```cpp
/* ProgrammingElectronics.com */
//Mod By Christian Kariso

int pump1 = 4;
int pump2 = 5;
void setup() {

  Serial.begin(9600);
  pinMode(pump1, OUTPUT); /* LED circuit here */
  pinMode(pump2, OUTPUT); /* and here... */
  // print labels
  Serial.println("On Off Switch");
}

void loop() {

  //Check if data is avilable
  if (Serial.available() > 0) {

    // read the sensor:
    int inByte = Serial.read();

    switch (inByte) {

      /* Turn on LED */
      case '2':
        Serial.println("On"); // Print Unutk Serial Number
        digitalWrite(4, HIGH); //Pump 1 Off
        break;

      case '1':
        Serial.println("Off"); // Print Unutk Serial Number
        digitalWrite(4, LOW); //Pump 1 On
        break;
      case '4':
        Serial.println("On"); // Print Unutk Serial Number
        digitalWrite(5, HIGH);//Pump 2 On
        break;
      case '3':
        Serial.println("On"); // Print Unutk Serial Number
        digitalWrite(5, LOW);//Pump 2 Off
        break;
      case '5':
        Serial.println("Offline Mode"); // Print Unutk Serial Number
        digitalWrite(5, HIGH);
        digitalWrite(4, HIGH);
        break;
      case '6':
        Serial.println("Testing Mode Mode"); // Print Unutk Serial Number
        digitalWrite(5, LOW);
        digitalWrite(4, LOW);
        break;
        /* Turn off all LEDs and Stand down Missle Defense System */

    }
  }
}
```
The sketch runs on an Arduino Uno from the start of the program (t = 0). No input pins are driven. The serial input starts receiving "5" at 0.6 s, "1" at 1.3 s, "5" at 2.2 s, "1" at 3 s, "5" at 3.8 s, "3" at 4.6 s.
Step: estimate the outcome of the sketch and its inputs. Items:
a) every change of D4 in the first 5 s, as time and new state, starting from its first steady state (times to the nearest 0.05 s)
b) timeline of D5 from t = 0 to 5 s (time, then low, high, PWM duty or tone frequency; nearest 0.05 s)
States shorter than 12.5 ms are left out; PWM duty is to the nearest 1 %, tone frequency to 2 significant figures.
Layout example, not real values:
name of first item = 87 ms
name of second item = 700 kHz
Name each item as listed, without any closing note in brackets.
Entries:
every change of D4 in the first 5 s, as time and new state, starting from its first steady state = 0 s low; 0.6 s high; 1.3 s low; 2.2 s high; 3 s low; 3.8 s high
timeline of D5 from t = 0 to 5 s = 0 s low; 0.6 s high; 4.6 s low
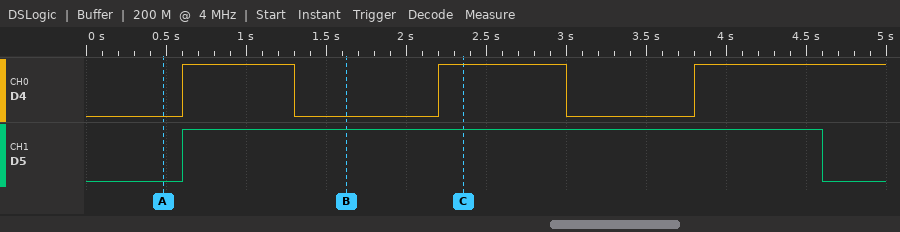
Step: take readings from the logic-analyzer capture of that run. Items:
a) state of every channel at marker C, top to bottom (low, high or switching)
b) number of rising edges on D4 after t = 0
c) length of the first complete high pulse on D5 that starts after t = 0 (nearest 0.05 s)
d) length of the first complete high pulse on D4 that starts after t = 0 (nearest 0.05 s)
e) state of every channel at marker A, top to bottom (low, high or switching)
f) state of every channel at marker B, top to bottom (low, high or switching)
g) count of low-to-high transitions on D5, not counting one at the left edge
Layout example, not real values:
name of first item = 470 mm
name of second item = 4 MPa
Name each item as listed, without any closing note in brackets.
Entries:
state of every channel at marker C, top to bottom = D4 high, D5 high
number of rising edges on D4 after t = 0 = 3
length of the first complete high pulse on D5 that starts after t = 0 = 4.00 s
length of the first complete high pulse on D4 that starts after t = 0 = 0.70 s
state of every channel at marker A, top to bottom = D4 low, D5 low
state of every channel at marker B, top to bottom = D4 low, D5 high
count of low-to-high transitions on D5, not counting one at the left edge = 1
